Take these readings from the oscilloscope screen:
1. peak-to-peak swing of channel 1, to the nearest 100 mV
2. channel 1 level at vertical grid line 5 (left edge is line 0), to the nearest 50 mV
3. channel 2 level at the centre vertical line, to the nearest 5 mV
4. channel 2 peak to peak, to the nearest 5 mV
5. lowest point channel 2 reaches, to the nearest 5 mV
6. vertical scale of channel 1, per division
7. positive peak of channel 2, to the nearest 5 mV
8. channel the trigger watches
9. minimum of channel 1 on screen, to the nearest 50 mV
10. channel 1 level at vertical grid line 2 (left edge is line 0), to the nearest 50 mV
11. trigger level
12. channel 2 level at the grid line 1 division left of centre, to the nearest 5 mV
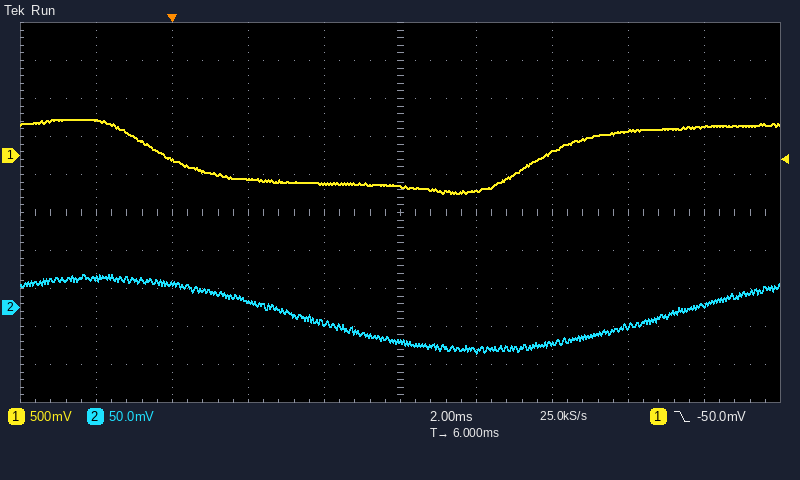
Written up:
1.00 V
-400 mV
-45 mV
105 mV
-60 mV
500 mV
45 mV
channel 1
-500 mV
-50 mV
-50.0 mV
-20 mV
